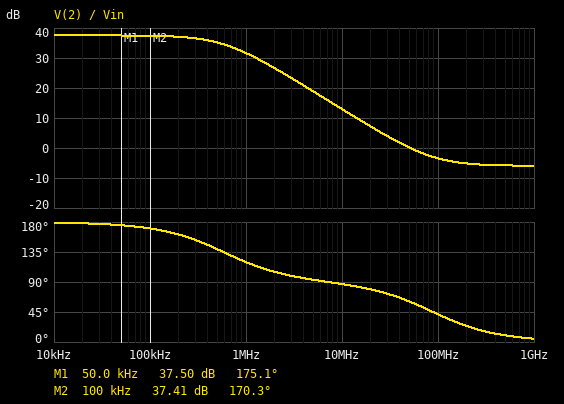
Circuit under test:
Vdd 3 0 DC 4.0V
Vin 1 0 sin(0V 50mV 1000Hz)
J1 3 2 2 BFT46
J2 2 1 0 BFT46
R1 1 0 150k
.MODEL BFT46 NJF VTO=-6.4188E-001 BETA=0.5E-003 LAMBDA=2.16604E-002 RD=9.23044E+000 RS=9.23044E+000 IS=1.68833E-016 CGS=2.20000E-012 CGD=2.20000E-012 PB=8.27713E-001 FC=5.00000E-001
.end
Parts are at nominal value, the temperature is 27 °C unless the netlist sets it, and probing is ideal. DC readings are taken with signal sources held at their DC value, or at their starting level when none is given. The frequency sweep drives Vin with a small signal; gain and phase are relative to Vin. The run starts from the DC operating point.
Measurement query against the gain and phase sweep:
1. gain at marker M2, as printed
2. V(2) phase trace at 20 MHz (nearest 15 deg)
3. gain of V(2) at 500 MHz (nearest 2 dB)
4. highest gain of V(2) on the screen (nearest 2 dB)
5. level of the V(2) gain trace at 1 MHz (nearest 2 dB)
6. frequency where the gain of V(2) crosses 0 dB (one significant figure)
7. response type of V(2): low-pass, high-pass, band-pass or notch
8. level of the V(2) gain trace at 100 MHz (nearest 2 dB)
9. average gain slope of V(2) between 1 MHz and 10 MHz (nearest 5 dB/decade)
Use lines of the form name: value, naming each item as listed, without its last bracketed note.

gain at marker M2, as printed: 37.41 dB
V(2) phase trace at 20 MHz: 75 deg
gain of V(2) at 500 MHz: -6 dB
highest gain of V(2) on the screen: 38 dB
level of the V(2) gain trace at 1 MHz: 32 dB
frequency where the gain of V(2) crosses 0 dB: 50 MHz
response type of V(2): low-pass, high-pass, band-pass or notch: low-pass
level of the V(2) gain trace at 100 MHz: -4 dB
average gain slope of V(2) between 1 MHz and 10 MHz: -20 dB/decade
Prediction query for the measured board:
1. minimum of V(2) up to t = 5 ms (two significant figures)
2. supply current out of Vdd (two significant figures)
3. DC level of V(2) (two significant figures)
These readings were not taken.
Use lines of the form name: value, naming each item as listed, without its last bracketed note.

minimum of V(2) up to t = 5 ms: 490 mV
supply current out of Vdd: 210 µA
DC level of V(2): 2.0 V
